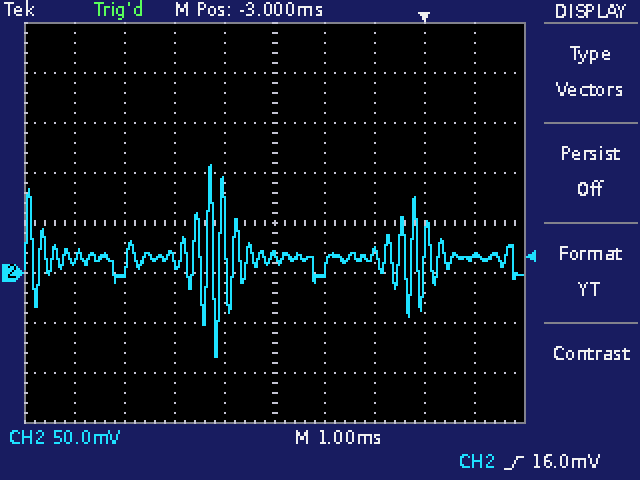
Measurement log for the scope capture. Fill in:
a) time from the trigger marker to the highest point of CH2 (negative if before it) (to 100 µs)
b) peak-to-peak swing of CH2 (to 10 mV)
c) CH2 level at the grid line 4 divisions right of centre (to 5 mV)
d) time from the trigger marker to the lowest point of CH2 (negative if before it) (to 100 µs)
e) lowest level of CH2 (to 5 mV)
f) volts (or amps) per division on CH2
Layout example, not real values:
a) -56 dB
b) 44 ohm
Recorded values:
a) -4.3 ms
b) 190 mV
c) 15 mV
d) -4.2 ms
e) -85 mV
f) 50 mV
